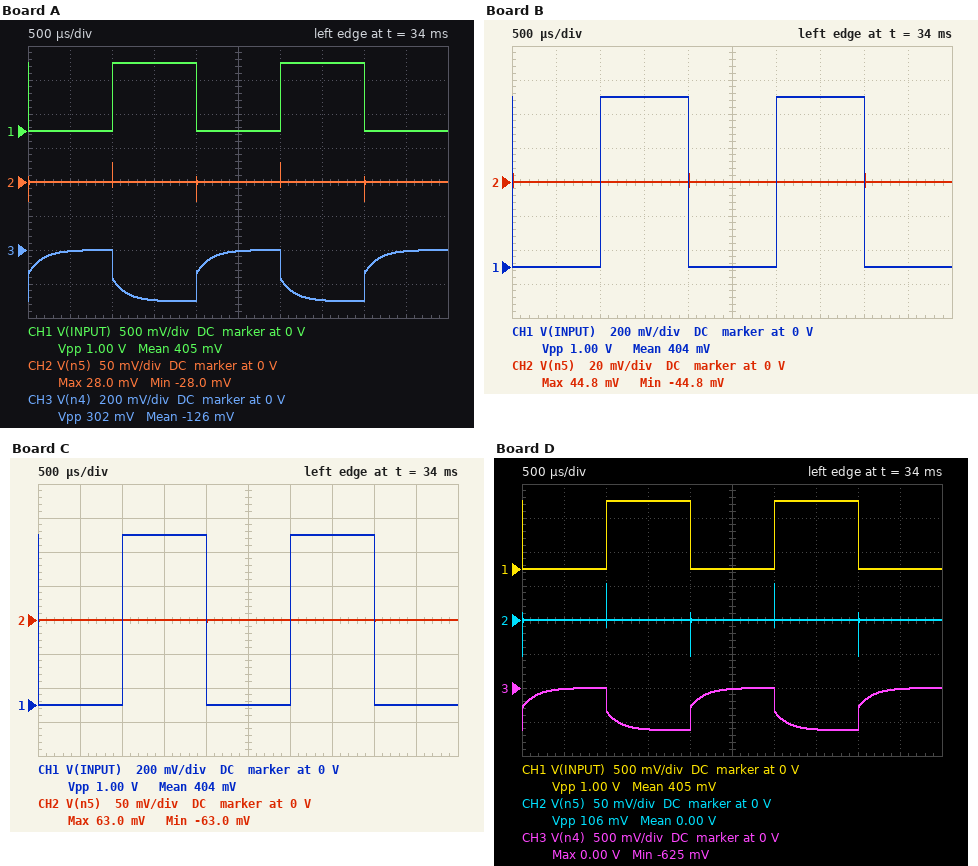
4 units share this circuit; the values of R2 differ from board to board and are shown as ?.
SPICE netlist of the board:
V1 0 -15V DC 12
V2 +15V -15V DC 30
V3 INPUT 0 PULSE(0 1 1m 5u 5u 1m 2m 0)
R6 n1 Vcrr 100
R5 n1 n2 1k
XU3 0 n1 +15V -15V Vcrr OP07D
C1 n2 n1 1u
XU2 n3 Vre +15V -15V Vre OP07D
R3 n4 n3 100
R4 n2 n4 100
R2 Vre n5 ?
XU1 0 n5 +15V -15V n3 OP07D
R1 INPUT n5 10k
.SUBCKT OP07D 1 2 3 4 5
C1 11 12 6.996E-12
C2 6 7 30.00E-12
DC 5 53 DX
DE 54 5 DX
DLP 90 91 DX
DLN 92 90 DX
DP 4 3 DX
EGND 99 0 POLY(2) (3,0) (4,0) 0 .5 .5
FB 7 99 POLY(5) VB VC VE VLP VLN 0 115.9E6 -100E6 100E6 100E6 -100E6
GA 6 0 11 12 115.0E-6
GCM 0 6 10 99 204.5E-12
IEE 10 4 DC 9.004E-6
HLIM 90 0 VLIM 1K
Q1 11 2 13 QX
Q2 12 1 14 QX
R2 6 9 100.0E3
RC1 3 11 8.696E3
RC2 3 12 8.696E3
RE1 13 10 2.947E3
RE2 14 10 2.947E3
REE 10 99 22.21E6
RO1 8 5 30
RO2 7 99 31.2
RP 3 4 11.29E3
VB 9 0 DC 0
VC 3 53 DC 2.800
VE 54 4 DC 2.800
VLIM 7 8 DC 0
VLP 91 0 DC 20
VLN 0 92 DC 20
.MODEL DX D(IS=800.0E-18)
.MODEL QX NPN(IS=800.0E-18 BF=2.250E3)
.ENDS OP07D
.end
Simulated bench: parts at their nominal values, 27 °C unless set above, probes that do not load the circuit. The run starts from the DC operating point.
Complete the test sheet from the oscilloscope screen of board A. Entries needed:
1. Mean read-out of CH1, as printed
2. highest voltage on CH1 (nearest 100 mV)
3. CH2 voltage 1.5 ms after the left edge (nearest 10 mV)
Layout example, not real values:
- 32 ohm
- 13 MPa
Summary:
- 405 mV
- 1.0 V
- 0 V
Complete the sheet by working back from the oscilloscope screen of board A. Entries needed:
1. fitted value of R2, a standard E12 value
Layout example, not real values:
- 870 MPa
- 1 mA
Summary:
- 3.3 kΩ
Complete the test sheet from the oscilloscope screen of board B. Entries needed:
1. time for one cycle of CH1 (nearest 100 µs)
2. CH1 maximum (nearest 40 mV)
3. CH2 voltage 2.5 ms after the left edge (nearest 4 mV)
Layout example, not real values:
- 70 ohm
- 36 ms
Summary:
- 2.0 ms
- 1.00 V
- 0 V
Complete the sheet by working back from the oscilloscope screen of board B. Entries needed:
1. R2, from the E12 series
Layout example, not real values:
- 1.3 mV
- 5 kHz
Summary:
- 5.6 kΩ
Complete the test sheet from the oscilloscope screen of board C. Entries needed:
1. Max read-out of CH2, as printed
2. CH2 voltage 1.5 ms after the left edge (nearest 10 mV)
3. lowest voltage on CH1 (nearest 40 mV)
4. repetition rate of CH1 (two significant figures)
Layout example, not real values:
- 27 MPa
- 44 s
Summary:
- 63.0 mV
- 0 V
- 0 V
- 500 Hz
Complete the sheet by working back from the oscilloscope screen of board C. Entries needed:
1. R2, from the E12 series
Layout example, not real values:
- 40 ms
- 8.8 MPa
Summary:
- 8.2 kΩ
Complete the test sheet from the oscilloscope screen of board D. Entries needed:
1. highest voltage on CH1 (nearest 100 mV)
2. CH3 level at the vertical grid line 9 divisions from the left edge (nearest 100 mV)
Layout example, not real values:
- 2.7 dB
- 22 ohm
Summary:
- 1.0 V
- 0 V
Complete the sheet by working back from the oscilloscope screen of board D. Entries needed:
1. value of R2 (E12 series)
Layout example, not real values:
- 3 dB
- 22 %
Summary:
- 6.8 kΩ
